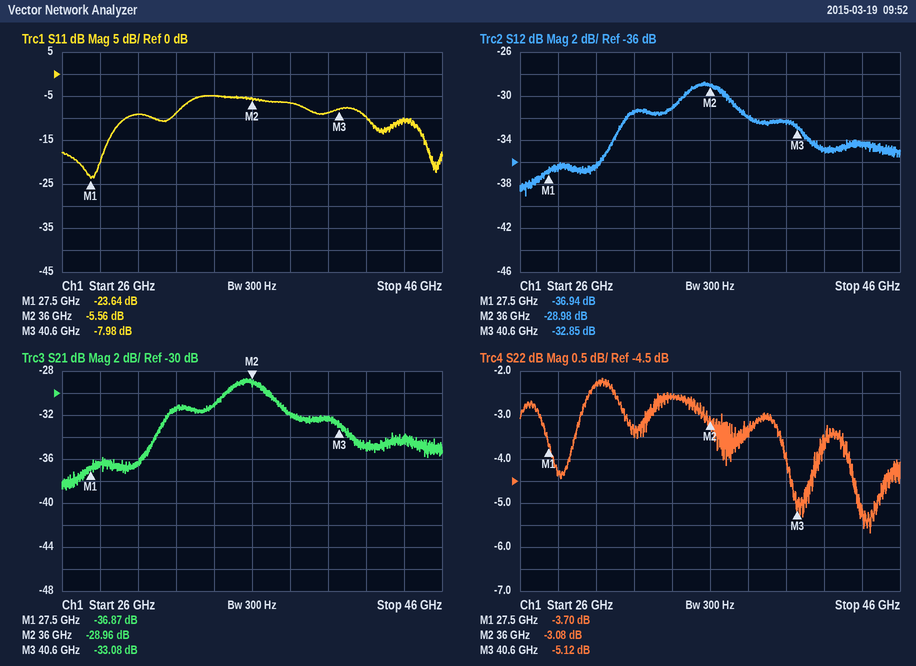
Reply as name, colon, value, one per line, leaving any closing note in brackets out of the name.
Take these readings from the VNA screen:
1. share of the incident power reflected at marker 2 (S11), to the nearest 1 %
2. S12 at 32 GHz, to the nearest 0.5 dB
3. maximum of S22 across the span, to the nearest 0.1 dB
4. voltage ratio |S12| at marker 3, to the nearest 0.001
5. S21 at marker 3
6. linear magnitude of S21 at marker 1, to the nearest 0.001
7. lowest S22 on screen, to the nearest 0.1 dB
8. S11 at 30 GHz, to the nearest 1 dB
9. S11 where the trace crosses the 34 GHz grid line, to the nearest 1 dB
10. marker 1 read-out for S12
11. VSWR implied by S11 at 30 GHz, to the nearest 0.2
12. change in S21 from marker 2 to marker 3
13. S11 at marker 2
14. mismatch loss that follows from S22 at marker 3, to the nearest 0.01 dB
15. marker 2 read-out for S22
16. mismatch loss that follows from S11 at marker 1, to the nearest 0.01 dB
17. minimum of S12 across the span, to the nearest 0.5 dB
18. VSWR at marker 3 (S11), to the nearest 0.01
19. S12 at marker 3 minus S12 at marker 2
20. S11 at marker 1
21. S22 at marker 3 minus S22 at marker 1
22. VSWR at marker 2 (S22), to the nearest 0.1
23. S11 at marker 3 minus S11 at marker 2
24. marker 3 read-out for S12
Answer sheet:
share of the incident power reflected at marker 2 (S11), to the nearest 1 %: 28 %
S12 at 32 GHz, to the nearest 0.5 dB: -31.5 dB
maximum of S22 across the span, to the nearest 0.1 dB: -2.2 dB
voltage ratio |S12| at marker 3, to the nearest 0.001: 0.023
S21 at marker 3: -33.08 dB
linear magnitude of S21 at marker 1, to the nearest 0.001: 0.014
lowest S22 on screen, to the nearest 0.1 dB: -5.7 dB
S11 at 30 GHz, to the nearest 1 dB: -9 dB
S11 where the trace crosses the 34 GHz grid line, to the nearest 1 dB: -5 dB
marker 1 read-out for S12: -36.94 dB
VSWR implied by S11 at 30 GHz, to the nearest 0.2: 2.0
change in S21 from marker 2 to marker 3: -4.12 dB
S11 at marker 2: -5.56 dB
mismatch loss that follows from S22 at marker 3, to the nearest 0.01 dB: 1.60 dB
marker 2 read-out for S22: -3.08 dB
mismatch loss that follows from S11 at marker 1, to the nearest 0.01 dB: 0.02 dB
minimum of S12 across the span, to the nearest 0.5 dB: -39.0 dB
VSWR at marker 3 (S11), to the nearest 0.01: 2.33
S12 at marker 3 minus S12 at marker 2: -3.87 dB
S11 at marker 1: -23.64 dB
S22 at marker 3 minus S22 at marker 1: -1.42 dB
VSWR at marker 2 (S22), to the nearest 0.1: 5.7
S11 at marker 3 minus S11 at marker 2: -2.42 dB
marker 3 read-out for S12: -32.85 dB
